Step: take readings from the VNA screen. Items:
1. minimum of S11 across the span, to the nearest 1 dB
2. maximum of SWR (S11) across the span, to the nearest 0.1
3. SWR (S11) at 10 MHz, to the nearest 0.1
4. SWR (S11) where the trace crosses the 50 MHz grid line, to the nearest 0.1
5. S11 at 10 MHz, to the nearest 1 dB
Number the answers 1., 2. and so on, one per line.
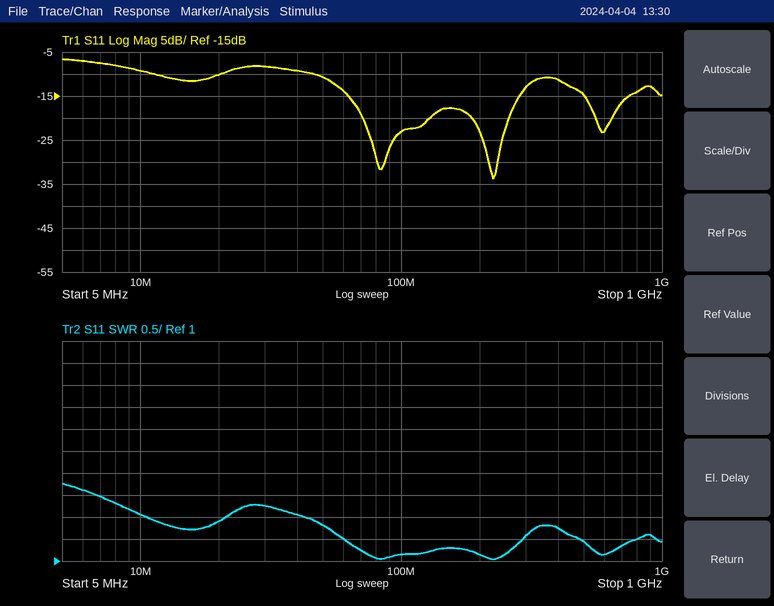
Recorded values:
1. -34 dB
2. 2.8
3. 2.1
4. 1.8
5. -9 dB
